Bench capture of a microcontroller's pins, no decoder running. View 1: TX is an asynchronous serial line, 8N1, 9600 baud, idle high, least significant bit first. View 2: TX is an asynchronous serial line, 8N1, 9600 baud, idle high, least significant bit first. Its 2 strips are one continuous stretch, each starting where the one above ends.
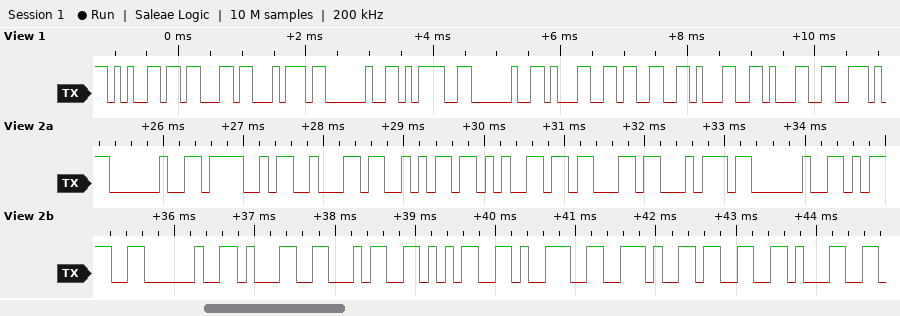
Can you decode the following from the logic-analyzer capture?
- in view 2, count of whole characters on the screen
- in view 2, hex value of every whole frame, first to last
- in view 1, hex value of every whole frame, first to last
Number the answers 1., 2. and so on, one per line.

1. 17
2. 20 4F 62 6A 65 63 74 20 3D 20 31 34 35 39 2E 33 31
3. 65 63 74 20 3D 20 31 33 31 31
